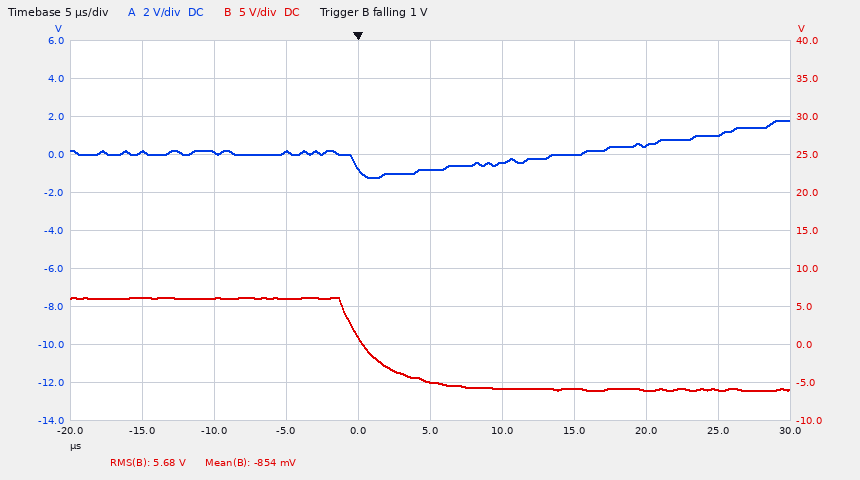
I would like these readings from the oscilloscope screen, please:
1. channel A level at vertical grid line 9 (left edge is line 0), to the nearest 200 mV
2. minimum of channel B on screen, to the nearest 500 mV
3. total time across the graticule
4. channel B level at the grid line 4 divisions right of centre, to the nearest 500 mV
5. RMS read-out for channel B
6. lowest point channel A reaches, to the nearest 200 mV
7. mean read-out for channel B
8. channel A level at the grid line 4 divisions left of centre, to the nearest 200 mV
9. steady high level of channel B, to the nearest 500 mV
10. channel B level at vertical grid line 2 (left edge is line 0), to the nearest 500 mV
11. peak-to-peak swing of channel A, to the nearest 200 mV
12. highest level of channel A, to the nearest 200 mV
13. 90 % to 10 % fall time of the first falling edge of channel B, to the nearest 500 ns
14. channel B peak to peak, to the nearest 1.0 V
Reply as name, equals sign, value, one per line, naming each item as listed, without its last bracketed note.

channel A level at vertical grid line 9 (left edge is line 0), to the nearest 200 mV = 1.0 V
minimum of channel B on screen, to the nearest 500 mV = -6.0 V
total time across the graticule = 50 µs
channel B level at the grid line 4 divisions right of centre, to the nearest 500 mV = -6.0 V
RMS read-out for channel B = 5.68 V
lowest point channel A reaches, to the nearest 200 mV = -1.2 V
mean read-out for channel B = -854 mV
channel A level at the grid line 4 divisions left of centre, to the nearest 200 mV = 200 mV
steady high level of channel B, to the nearest 500 mV = 6.0 V
channel B level at vertical grid line 2 (left edge is line 0), to the nearest 500 mV = 6.0 V
peak-to-peak swing of channel A, to the nearest 200 mV = 3.0 V
highest level of channel A, to the nearest 200 mV = 1.8 V
90 % to 10 % fall time of the first falling edge of channel B, to the nearest 500 ns = 5.5 µs
channel B peak to peak, to the nearest 1.0 V = 12.0 V
